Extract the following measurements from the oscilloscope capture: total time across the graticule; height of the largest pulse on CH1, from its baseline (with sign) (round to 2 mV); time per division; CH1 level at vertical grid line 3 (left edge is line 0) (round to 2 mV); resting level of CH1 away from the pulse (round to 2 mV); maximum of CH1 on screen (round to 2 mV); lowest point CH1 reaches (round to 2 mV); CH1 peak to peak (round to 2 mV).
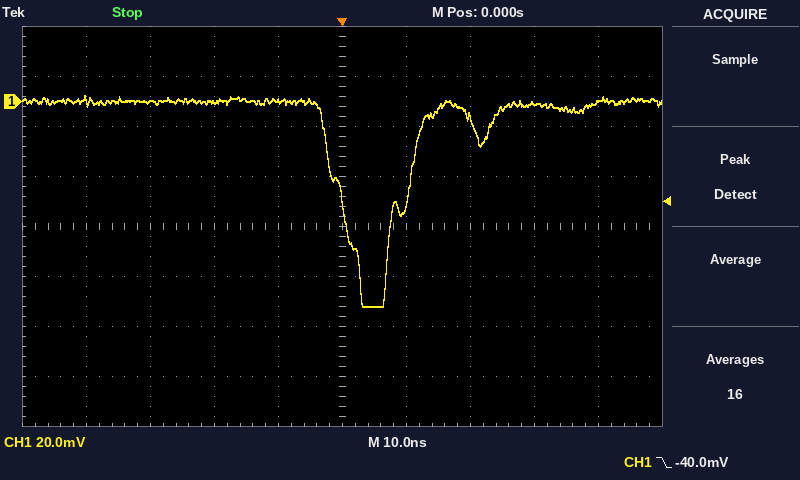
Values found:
100 ns
-82 mV
10 ns
0 mV
0 mV
2 mV
-82 mV
84 mV
